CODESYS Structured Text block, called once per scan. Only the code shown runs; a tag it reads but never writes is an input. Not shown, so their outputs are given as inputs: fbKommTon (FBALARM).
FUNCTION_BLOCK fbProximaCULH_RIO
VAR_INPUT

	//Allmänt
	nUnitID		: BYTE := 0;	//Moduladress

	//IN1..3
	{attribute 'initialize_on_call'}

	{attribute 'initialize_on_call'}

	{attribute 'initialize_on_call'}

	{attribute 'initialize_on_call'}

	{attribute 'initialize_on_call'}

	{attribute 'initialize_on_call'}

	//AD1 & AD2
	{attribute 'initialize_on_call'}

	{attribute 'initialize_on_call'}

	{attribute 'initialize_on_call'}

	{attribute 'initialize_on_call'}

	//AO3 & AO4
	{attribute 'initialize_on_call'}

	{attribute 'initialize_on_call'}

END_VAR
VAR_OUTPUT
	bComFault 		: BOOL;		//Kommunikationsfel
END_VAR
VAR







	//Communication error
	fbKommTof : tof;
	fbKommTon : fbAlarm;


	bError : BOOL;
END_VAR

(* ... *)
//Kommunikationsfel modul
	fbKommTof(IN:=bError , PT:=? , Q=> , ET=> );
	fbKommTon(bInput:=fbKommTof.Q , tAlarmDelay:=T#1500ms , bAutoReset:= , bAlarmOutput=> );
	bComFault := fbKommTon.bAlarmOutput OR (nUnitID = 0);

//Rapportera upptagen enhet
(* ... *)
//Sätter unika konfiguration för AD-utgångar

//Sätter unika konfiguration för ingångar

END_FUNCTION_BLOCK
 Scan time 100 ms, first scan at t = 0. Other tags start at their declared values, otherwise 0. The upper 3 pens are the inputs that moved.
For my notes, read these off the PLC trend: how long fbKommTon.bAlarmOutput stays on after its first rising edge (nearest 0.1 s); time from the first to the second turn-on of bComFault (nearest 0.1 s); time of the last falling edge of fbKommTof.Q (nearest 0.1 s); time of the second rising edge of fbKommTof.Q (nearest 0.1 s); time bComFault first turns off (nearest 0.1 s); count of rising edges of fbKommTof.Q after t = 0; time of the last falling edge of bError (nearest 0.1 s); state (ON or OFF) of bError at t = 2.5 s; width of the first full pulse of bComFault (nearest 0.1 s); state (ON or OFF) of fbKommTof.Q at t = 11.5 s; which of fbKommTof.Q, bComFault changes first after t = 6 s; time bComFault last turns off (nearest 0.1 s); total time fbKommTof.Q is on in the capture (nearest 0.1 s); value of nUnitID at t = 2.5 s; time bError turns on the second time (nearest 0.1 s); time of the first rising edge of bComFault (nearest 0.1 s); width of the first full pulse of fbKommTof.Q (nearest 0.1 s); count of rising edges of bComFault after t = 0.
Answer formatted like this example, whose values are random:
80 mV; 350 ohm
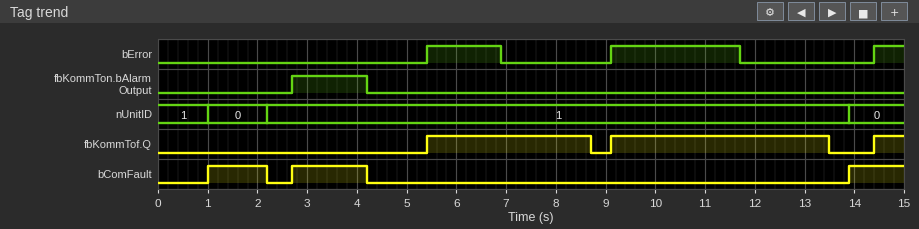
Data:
1.5 s; 1.7 s; 13.5 s; 9.1 s; 2.2 s; 3; 11.7 s; OFF; 1.2 s; ON; fbKommTof.Q; 4.2 s; 8.3 s; 1; 9.1 s; 1.0 s; 3.3 s; 3
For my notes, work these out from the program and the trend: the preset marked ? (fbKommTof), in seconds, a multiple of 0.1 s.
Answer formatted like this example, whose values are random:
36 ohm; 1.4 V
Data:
1.8 s
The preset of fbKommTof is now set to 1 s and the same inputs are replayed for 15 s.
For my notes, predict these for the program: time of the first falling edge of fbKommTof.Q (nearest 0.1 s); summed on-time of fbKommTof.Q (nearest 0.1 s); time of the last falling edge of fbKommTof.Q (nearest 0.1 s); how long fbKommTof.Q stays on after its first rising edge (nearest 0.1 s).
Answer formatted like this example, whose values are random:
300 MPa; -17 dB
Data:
7.9 s; 6.7 s; 12.7 s; 2.5 s
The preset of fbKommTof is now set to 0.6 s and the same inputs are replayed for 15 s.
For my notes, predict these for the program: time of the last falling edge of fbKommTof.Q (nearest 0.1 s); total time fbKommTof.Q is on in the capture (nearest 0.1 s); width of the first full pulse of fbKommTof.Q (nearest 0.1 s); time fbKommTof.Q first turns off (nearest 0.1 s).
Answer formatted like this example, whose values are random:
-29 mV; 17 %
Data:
12.3 s; 5.9 s; 2.1 s; 7.5 s
